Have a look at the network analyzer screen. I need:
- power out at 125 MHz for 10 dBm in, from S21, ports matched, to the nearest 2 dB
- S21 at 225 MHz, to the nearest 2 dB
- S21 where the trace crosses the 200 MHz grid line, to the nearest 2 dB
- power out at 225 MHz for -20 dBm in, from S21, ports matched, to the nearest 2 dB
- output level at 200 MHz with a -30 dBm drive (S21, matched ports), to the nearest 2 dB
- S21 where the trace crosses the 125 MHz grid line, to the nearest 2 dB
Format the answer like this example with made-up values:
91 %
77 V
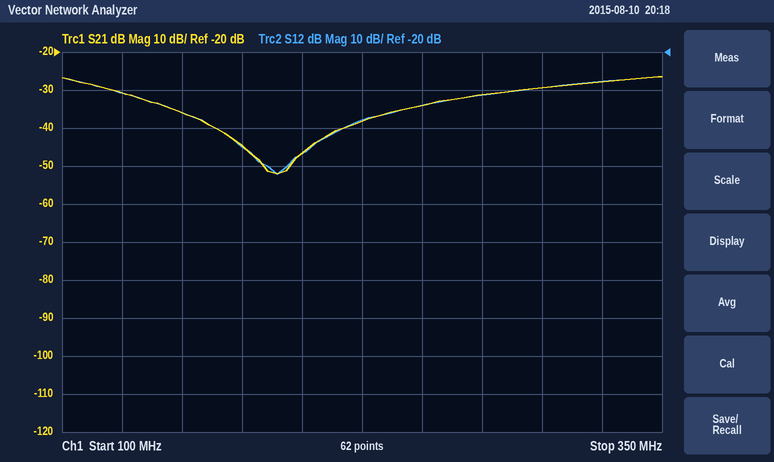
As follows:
-20 dBm
-38 dB
-46 dB
-58 dBm
-76 dBm
-30 dB
